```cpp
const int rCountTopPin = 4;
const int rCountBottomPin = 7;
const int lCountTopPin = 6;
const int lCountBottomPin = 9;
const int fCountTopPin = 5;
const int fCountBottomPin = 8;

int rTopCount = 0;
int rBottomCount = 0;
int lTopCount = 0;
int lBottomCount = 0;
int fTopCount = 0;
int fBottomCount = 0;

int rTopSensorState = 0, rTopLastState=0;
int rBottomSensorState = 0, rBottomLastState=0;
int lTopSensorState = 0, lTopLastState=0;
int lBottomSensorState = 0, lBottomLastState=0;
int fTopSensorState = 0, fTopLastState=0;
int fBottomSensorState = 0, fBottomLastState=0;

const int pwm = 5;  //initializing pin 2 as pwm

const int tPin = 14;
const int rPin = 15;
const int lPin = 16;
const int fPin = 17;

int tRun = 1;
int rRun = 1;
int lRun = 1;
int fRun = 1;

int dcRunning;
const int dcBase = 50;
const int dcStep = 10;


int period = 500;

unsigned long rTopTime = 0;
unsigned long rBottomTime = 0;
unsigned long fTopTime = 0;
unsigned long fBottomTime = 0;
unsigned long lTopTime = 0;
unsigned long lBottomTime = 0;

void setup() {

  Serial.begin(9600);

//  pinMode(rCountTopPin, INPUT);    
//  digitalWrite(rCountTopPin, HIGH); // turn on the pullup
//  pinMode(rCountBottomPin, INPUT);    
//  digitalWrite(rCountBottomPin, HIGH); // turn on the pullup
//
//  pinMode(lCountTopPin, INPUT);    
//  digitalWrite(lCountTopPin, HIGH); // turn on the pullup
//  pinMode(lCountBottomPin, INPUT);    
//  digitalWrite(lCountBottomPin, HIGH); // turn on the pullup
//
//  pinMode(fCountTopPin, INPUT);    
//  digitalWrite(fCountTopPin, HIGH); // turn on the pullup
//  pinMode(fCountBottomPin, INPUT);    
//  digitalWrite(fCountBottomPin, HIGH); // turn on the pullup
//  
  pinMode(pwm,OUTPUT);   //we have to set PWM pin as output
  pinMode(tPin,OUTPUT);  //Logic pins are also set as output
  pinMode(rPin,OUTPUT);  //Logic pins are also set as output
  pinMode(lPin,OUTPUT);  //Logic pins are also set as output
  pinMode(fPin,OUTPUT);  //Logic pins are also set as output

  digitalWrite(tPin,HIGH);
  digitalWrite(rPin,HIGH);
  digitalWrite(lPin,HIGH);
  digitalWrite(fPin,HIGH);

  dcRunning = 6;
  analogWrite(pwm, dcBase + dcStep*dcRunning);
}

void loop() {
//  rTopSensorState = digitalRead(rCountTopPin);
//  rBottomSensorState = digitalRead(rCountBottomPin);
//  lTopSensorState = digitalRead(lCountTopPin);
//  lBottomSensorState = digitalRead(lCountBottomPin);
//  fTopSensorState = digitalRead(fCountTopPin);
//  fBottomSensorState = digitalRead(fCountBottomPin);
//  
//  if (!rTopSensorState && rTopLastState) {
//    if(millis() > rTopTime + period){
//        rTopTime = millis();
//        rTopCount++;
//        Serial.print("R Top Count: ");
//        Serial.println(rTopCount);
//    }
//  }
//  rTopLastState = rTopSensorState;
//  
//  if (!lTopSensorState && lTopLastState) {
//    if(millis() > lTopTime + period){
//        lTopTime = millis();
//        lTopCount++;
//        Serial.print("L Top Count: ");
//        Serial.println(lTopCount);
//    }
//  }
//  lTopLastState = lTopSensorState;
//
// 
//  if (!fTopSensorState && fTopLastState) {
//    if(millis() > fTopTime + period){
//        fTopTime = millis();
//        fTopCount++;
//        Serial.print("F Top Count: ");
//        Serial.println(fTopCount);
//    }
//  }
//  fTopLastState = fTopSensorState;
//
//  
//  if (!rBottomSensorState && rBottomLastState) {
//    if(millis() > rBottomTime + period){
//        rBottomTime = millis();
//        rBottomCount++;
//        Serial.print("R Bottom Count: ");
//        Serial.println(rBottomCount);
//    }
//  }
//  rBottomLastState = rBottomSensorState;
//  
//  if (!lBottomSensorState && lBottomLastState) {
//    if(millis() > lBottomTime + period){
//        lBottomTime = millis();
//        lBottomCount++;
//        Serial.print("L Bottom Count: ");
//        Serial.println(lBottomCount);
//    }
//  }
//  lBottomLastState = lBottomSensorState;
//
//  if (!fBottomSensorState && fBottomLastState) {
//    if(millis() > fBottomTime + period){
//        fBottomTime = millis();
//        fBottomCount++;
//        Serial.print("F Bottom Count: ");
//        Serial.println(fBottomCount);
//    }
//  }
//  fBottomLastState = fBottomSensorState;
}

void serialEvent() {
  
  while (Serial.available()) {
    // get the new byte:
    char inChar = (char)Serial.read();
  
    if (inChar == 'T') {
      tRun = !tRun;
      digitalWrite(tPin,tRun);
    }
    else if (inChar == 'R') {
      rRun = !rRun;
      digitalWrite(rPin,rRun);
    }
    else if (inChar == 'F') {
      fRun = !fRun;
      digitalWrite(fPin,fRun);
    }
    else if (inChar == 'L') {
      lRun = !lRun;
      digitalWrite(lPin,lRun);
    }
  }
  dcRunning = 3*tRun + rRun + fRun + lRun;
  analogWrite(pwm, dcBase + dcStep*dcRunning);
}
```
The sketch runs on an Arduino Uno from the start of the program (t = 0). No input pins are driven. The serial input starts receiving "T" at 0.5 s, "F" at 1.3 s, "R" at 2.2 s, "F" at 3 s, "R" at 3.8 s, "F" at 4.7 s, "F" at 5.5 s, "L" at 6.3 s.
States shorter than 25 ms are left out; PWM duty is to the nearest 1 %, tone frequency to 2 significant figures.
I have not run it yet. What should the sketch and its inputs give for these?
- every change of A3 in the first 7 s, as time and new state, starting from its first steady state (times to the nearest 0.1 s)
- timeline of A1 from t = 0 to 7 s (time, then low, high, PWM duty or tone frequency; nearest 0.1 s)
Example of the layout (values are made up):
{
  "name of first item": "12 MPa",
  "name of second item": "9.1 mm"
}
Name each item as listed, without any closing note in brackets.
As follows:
{
  "every change of A3 in the first 7 s, as time and new state, starting from its first steady state": "0 s high; 1.3 s low; 3 s high; 4.7 s low; 5.5 s high",
  "timeline of A1 from t = 0 to 7 s": "0 s high; 2.2 s low; 3.8 s high"
}
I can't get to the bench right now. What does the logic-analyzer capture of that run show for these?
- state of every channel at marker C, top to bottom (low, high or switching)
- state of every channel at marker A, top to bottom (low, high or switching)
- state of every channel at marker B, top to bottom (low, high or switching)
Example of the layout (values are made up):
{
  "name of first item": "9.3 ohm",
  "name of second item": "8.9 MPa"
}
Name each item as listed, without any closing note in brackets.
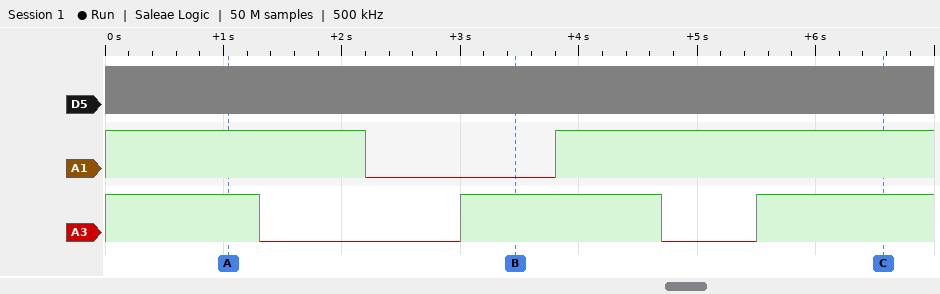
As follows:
{
  "state of every channel at marker C, top to bottom": "D5 switching, A1 high, A3 high",
  "state of every channel at marker A, top to bottom": "D5 switching, A1 high, A3 high",
  "state of every channel at marker B, top to bottom": "D5 switching, A1 low, A3 high"
}
